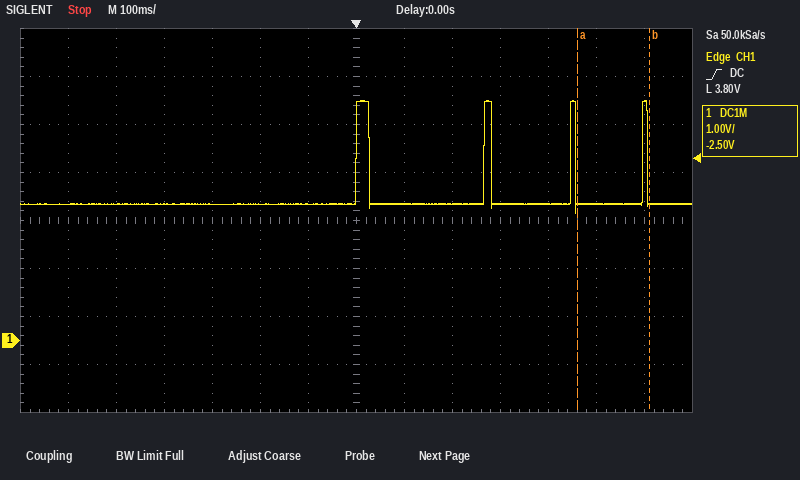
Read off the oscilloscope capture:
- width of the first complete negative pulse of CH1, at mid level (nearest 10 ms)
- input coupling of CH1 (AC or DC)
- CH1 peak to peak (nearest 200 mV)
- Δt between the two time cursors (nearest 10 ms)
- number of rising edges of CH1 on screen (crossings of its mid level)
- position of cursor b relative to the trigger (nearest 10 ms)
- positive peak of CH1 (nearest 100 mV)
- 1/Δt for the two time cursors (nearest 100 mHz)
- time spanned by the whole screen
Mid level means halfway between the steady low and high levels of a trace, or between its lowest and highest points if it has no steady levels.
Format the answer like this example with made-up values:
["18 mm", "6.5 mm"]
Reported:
["240 ms", "DC", "2.4 V", "150 ms", "4", "+610 ms", "5.0 V", "6.7 Hz", "1.4 s"]
